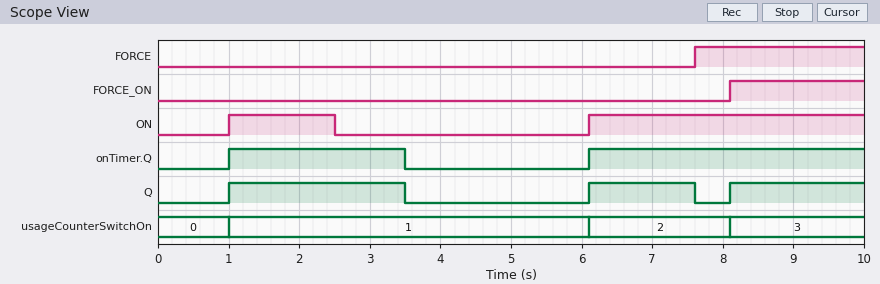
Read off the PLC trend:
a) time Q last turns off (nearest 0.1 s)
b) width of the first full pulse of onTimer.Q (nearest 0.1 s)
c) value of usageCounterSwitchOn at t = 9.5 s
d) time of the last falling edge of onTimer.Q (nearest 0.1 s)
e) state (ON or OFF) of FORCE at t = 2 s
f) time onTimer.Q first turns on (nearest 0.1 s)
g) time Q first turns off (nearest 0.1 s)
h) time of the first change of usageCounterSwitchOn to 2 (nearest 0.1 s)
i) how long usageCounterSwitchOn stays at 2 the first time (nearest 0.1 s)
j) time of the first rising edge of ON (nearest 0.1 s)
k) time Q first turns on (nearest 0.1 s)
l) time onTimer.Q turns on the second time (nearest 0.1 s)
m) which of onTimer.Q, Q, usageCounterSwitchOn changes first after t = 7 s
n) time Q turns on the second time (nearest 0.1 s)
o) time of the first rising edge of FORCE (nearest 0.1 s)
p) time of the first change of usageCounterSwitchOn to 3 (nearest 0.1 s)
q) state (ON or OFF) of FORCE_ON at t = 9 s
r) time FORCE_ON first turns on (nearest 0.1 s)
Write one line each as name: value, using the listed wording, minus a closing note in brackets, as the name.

time Q last turns off: 7.6 s
width of the first full pulse of onTimer.Q: 2.5 s
value of usageCounterSwitchOn at t = 9.5 s: 3
time of the last falling edge of onTimer.Q: 3.5 s
state (ON or OFF) of FORCE at t = 2 s: OFF
time onTimer.Q first turns on: 1.0 s
time Q first turns off: 3.5 s
time of the first change of usageCounterSwitchOn to 2: 6.1 s
how long usageCounterSwitchOn stays at 2 the first time: 2.0 s
time of the first rising edge of ON: 1.0 s
time Q first turns on: 1.0 s
time onTimer.Q turns on the second time: 6.1 s
which of onTimer.Q, Q, usageCounterSwitchOn changes first after t = 7 s: Q
time Q turns on the second time: 6.1 s
time of the first rising edge of FORCE: 7.6 s
time of the first change of usageCounterSwitchOn to 3: 8.1 s
state (ON or OFF) of FORCE_ON at t = 9 s: ON
time FORCE_ON first turns on: 8.1 s
